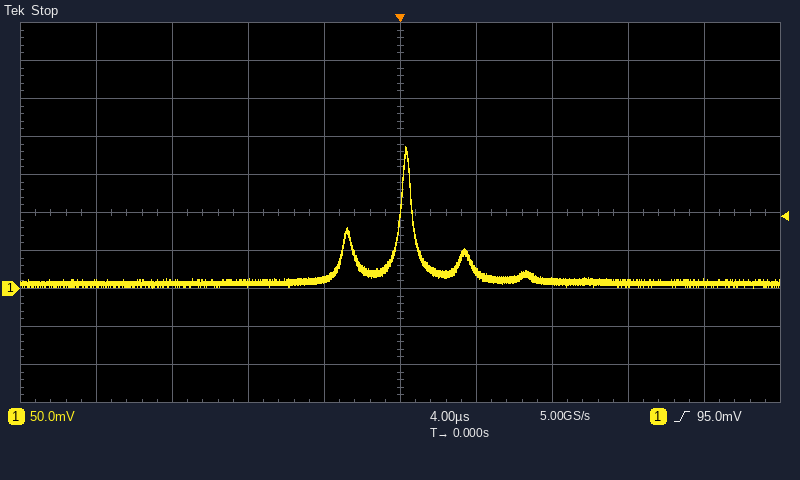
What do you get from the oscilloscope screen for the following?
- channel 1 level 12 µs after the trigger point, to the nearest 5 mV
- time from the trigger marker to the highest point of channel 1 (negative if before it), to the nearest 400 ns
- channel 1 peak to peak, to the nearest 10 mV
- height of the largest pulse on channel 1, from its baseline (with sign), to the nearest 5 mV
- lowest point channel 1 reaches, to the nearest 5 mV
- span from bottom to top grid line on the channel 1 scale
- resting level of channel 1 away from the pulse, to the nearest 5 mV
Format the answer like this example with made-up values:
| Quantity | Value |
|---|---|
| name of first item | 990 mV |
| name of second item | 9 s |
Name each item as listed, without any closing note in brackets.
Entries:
| Quantity | Value |
|---|---|
| channel 1 level 12 µs after the trigger point, to the nearest 5 mV | 5 mV |
| time from the trigger marker to the highest point of channel 1 (negative if before it), to the nearest 400 ns | +400 ns |
| channel 1 peak to peak, to the nearest 10 mV | 190 mV |
| height of the largest pulse on channel 1, from its baseline (with sign), to the nearest 5 mV | +180 mV |
| lowest point channel 1 reaches, to the nearest 5 mV | 0 mV |
| span from bottom to top grid line on the channel 1 scale | 500 mV |
| resting level of channel 1 away from the pulse, to the nearest 5 mV | 5 mV |
